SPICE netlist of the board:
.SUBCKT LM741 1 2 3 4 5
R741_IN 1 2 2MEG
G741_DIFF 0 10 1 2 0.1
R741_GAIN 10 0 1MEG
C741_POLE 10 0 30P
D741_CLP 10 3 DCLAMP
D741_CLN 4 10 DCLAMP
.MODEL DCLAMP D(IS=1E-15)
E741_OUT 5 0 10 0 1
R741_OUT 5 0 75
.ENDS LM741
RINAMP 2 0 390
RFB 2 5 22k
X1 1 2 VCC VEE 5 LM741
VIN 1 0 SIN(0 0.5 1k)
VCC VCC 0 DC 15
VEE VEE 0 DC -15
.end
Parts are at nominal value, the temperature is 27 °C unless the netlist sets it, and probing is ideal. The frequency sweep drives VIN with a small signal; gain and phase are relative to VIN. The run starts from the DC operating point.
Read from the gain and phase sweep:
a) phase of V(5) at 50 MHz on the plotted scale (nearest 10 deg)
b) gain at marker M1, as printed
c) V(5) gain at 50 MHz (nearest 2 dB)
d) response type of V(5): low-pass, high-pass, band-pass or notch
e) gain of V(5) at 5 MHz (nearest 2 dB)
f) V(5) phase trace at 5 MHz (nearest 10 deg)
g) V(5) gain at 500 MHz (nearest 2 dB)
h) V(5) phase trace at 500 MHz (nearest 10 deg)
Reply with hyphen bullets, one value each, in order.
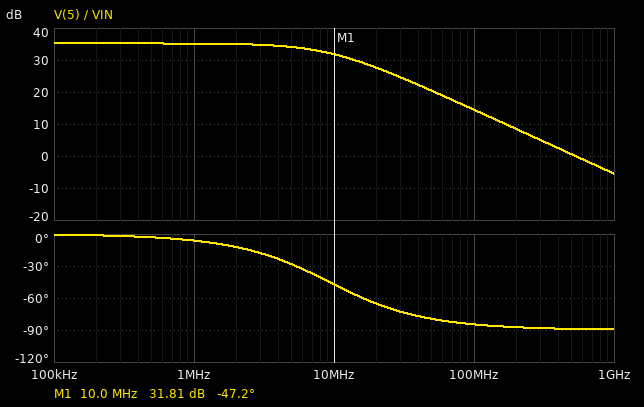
- -80 deg
- 31.81 dB
- 20 dB
- low-pass
- 34 dB
- -30 deg
- 0 dB
- -90 deg
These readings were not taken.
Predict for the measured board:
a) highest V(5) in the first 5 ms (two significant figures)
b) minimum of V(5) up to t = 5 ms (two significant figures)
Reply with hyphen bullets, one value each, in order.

- 16 V
- -16 V
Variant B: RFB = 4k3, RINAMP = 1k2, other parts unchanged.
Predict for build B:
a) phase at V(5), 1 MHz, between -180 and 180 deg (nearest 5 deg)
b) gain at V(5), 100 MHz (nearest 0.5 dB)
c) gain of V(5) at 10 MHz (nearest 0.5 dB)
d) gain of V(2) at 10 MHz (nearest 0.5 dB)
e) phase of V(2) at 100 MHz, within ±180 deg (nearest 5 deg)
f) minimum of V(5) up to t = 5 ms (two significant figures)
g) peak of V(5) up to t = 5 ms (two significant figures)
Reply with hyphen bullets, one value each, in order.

- 0 deg
- 11.0 dB
- 13.0 dB
- 0 dB
- -40 deg
- -2.3 V
- 2.3 V
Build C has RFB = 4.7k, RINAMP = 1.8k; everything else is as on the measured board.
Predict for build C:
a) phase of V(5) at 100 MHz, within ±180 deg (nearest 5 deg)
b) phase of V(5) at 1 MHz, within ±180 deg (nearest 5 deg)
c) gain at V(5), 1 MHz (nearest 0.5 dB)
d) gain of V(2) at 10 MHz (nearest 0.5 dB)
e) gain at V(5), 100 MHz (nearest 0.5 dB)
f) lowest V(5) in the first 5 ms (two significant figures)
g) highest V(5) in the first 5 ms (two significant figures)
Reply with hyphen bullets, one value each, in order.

- -35 deg
- 0 deg
- 11.0 dB
- 0 dB
- 9.5 dB
- -1.8 V
- 1.8 V
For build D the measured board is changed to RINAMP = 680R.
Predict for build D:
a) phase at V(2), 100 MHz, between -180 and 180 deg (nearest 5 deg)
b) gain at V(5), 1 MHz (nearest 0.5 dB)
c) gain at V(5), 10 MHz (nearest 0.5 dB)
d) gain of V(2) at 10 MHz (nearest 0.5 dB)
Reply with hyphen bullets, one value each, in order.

- -80 deg
- 30.5 dB
- 29.0 dB
- -1.5 dB
